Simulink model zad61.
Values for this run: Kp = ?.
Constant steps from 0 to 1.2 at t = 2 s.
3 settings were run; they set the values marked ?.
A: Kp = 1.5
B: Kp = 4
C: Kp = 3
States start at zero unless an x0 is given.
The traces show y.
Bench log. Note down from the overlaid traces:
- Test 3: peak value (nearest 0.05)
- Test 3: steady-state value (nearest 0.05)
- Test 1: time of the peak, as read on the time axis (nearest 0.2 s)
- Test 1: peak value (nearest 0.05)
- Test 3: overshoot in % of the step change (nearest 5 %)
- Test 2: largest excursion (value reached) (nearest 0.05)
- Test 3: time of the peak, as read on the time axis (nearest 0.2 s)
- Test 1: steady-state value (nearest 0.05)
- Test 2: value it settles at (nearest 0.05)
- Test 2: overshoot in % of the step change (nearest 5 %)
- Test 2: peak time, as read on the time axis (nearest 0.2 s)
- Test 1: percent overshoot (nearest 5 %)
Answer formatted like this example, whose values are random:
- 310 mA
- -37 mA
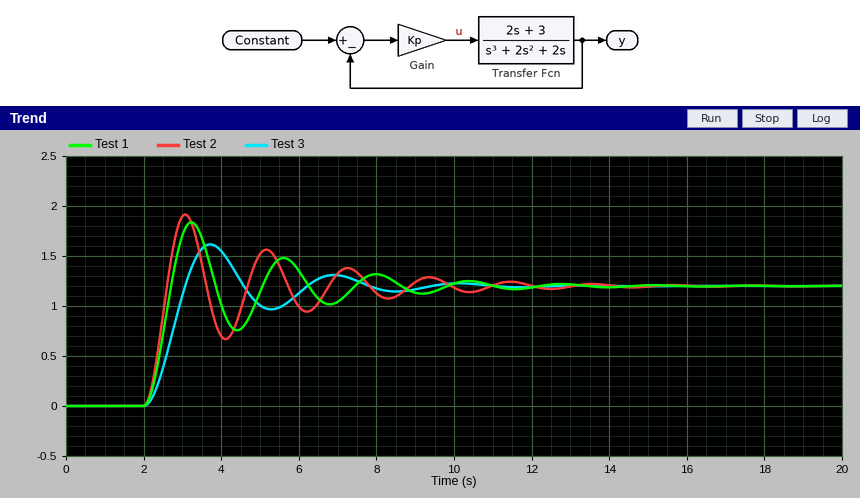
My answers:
- 1.60
- 1.20
- 3.2 s
- 1.85
- 35 %
- 1.90
- 3.8 s
- 1.20
- 1.20
- 60 %
- 3.0 s
- 55 %
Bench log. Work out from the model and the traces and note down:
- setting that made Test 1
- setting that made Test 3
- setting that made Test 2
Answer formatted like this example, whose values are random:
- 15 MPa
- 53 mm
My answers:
- C
- A
- B
